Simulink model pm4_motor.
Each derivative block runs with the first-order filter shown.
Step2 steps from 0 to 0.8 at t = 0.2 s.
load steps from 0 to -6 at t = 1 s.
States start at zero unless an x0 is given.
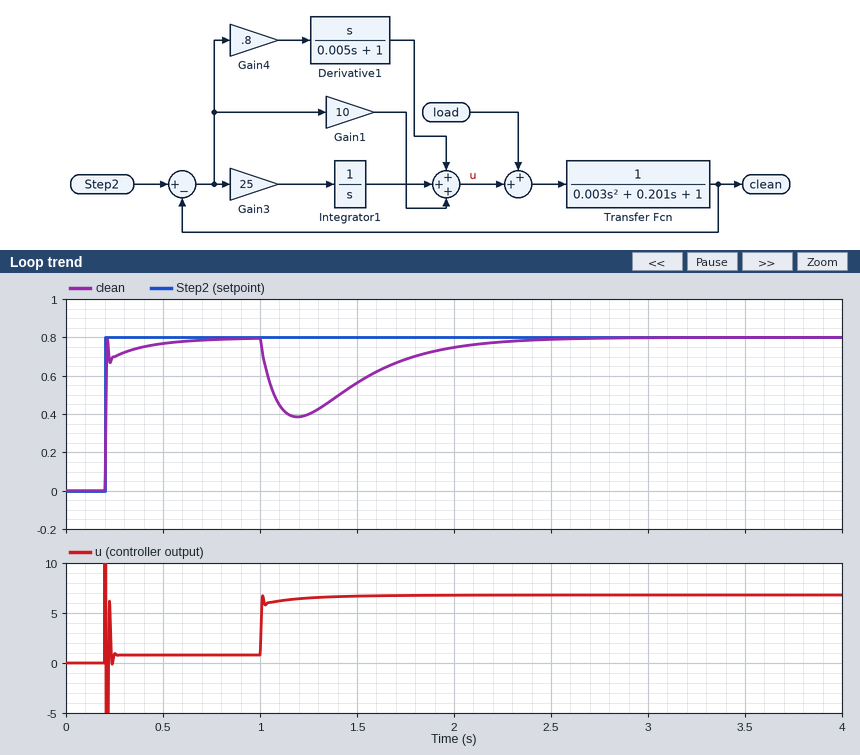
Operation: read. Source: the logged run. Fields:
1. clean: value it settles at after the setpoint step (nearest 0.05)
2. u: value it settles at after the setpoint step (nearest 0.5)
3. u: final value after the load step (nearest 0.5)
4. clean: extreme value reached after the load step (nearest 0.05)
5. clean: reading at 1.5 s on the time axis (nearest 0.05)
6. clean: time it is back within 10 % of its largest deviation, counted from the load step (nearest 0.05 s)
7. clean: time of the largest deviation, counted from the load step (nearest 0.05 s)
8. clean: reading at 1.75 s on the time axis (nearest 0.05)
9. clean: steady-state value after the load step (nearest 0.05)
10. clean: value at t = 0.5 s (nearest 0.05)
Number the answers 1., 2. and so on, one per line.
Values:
1. 0.80
2. 1.0
3. 7.0
4. 0.40
5. 0.55
6. 1.10 s
7. 0.20 s
8. 0.70
9. 0.80
10. 0.75
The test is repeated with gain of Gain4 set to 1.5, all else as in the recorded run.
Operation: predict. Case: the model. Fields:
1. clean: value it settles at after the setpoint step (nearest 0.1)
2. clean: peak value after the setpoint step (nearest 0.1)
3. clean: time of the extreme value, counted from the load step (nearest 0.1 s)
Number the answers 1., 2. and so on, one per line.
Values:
1. 0.8
2. 0.9
3. 0.3 s
